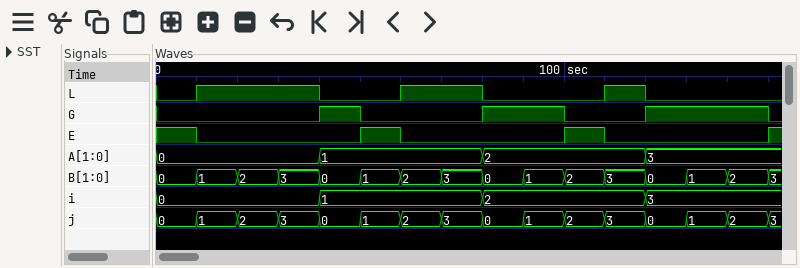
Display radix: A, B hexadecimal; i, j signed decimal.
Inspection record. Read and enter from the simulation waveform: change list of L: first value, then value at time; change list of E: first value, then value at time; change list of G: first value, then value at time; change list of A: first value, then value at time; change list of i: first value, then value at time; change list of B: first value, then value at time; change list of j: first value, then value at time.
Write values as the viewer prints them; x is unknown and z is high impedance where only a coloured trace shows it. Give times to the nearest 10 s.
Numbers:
0, 1 at 10 s, 0 at 40 s, 1 at 60 s, 0 at 80 s, 1 at 110 s, 0 at 120 s
1, 0 at 10 s, 1 at 50 s, 0 at 60 s, 1 at 100 s, 0 at 110 s, 1 at 150 s
0, 1 at 40 s, 0 at 50 s, 1 at 80 s, 0 at 100 s, 1 at 120 s, 0 at 150 s
0, 1 at 40 s, 2 at 80 s, 3 at 120 s
0, 1 at 40 s, 2 at 80 s, 3 at 120 s
0, 1 at 10 s, 2 at 20 s, 3 at 30 s, 0 at 40 s, 1 at 50 s, 2 at 60 s, 3 at 70 s, 0 at 80 s, 1 at 90 s, 2 at 100 s, 3 at 110 s, 0 at 120 s, 1 at 130 s, 2 at 140 s, 3 at 150 s
0, 1 at 10 s, 2 at 20 s, 3 at 30 s, 0 at 40 s, 1 at 50 s, 2 at 60 s, 3 at 70 s, 0 at 80 s, 1 at 90 s, 2 at 100 s, 3 at 110 s, 0 at 120 s, 1 at 130 s, 2 at 140 s, 3 at 150 s
